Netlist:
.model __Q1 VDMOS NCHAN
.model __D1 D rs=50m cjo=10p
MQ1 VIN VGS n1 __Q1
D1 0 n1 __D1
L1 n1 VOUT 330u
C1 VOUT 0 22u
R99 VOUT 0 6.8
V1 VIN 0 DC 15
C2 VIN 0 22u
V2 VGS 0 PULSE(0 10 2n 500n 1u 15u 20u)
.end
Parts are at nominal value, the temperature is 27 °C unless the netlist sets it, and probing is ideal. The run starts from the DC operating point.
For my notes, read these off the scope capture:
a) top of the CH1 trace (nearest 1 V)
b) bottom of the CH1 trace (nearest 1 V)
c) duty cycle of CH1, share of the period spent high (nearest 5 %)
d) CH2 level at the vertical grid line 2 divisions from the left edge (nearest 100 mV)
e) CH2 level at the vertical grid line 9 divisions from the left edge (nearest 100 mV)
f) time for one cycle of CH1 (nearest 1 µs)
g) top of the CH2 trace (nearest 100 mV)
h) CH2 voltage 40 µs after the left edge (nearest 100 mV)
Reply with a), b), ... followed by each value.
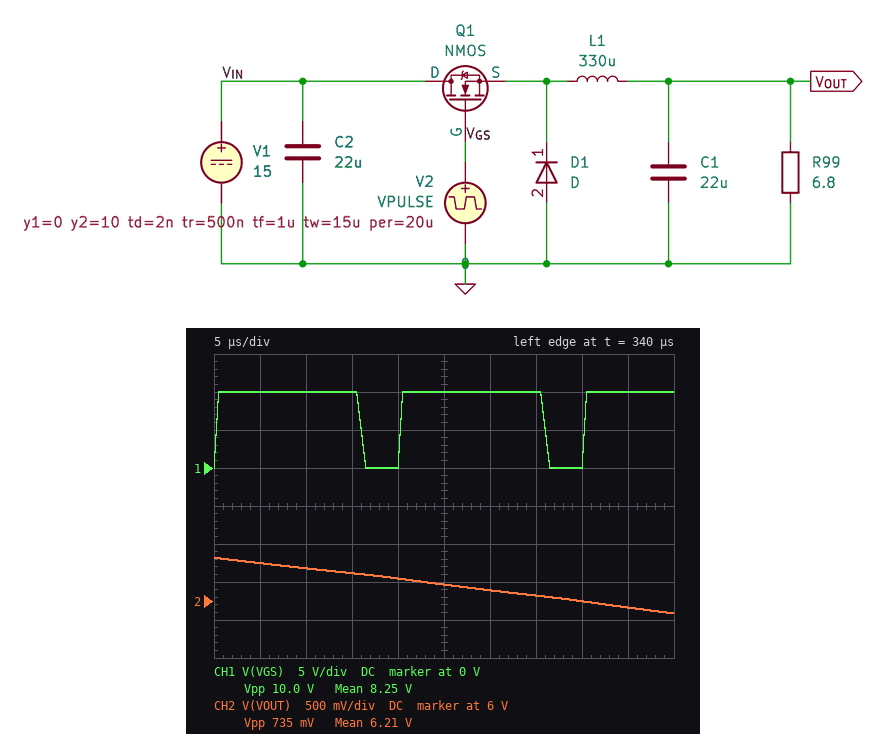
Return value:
a) 10 V
b) 0 V
c) 80 %
d) 6.4 V
e) 5.9 V
f) 20 µs
g) 6.6 V
h) 6.0 V
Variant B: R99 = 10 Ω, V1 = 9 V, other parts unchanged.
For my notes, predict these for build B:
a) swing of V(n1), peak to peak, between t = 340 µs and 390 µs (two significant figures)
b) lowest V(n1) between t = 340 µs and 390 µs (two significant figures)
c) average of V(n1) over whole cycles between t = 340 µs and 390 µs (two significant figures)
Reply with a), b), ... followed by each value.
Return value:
a) 7.8 V
b) -810 mV
c) 5.2 V
